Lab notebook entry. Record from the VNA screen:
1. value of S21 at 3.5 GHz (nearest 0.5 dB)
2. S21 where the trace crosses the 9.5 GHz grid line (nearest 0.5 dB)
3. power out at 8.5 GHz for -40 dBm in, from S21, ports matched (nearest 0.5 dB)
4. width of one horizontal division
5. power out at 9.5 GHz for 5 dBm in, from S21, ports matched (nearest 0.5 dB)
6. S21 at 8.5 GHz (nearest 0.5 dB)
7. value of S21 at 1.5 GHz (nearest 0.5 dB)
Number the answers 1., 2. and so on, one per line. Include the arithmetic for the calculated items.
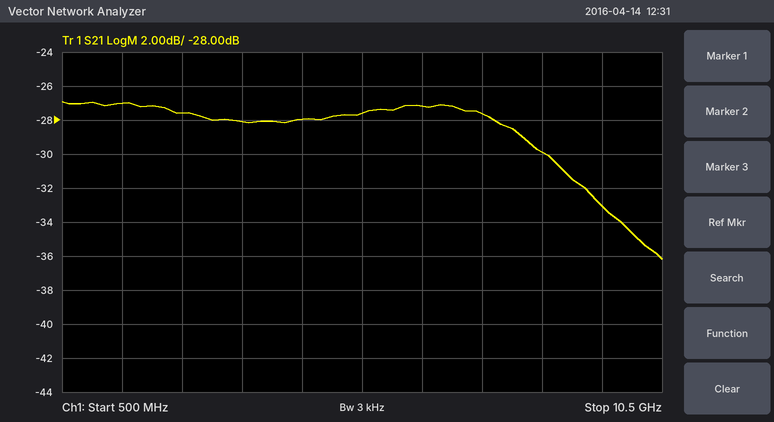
1. -28.0 dB
2. -33.0 dB
3. -40 dBm + (-30.0 dB) = -70.0 dBm
4. 1 GHz
5. 5 dBm + (-33.0 dB) = -28.0 dBm
6. -30.0 dB
7. -27.0 dB
